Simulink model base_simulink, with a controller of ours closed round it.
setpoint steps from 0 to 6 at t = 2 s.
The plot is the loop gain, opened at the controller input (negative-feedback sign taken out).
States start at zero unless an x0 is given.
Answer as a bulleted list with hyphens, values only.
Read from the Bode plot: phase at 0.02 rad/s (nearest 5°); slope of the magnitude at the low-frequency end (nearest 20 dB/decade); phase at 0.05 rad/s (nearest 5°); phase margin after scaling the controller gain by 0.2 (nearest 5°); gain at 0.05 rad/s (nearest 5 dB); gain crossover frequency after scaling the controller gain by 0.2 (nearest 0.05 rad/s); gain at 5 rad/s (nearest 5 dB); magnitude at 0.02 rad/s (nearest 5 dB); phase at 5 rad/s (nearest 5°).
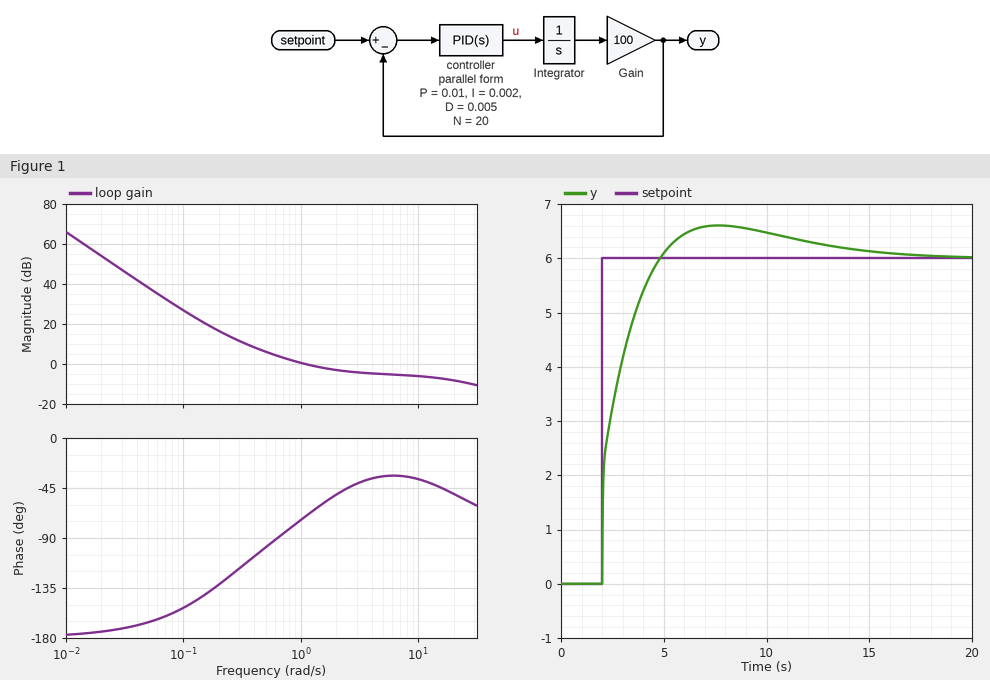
- -175°
- -40 dB/decade
- -165°
- 55°
- 40 dB
- 0.25 rad/s
- -5 dB
- 55 dB
- -35°
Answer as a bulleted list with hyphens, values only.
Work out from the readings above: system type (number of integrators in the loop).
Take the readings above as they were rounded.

- 2
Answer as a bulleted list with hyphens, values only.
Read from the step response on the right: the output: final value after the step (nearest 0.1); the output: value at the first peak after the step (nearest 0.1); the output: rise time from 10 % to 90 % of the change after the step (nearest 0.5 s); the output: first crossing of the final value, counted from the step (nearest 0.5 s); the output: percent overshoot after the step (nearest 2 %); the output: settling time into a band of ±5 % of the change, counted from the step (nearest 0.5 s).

- 6.0
- 6.6
- 2.0 s
- 3.0 s
- 10 %
- 10.0 s
